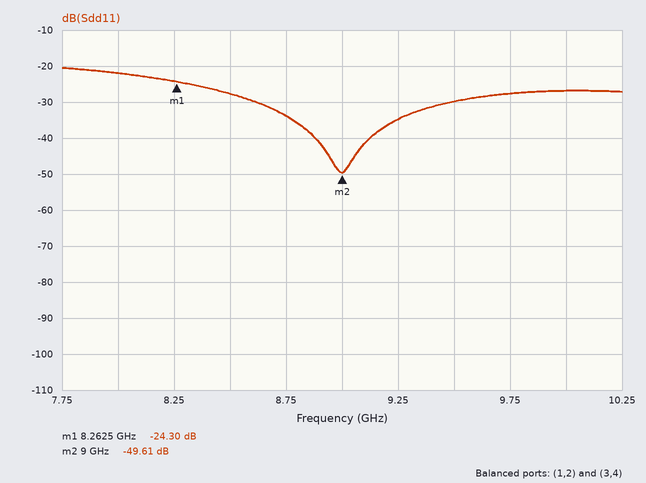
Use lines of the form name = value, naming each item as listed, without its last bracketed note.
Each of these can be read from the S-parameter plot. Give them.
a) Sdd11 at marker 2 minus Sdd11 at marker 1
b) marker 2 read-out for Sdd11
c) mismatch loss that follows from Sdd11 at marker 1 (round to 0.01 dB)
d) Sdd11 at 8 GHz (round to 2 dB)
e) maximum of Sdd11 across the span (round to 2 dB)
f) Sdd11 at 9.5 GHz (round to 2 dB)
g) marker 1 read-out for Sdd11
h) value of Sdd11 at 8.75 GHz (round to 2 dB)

Sdd11 at marker 2 minus Sdd11 at marker 1 = -25.31 dB
marker 2 read-out for Sdd11 = -49.61 dB
mismatch loss that follows from Sdd11 at marker 1 = 0.02 dB
Sdd11 at 8 GHz = -22 dB
maximum of Sdd11 across the span = -20 dB
Sdd11 at 9.5 GHz = -30 dB
marker 1 read-out for Sdd11 = -24.30 dB
value of Sdd11 at 8.75 GHz = -34 dB
